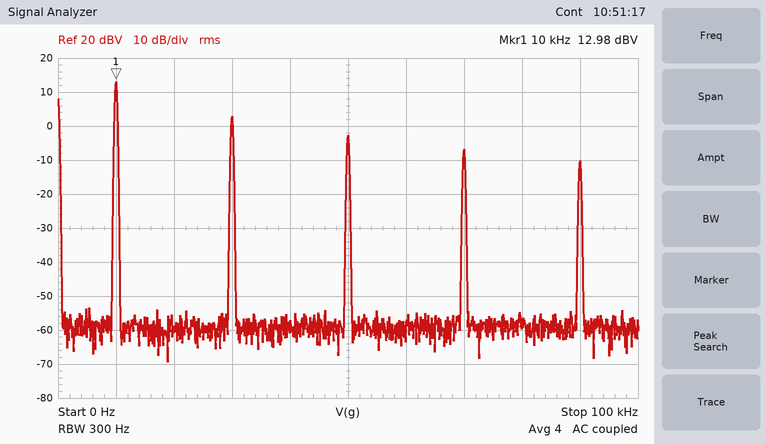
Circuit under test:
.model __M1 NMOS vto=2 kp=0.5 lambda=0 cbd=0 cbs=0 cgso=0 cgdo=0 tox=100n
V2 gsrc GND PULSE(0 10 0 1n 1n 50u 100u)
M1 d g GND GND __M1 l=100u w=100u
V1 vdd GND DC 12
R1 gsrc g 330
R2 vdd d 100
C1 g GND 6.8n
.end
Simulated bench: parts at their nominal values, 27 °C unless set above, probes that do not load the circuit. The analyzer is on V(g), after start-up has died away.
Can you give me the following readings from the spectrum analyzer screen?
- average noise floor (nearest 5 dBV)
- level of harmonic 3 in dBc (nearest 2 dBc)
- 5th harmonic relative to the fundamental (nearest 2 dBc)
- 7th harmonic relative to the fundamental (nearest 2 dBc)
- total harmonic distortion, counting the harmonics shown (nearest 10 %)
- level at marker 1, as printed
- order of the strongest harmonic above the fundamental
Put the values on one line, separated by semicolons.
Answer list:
-60 dBV; -10 dBc; -16 dBc; -20 dBc; 40 %; 12.98 dBV; 3
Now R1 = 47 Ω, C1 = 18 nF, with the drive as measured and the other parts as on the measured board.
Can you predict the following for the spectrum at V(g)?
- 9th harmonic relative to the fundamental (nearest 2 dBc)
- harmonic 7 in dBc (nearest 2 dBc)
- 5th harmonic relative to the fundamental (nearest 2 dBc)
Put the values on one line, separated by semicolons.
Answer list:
-20 dBc; -18 dBc; -14 dBc
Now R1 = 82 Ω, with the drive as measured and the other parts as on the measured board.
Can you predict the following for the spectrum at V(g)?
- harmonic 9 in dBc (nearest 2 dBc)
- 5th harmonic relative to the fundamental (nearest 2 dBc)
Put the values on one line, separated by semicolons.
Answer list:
-20 dBc; -14 dBc
